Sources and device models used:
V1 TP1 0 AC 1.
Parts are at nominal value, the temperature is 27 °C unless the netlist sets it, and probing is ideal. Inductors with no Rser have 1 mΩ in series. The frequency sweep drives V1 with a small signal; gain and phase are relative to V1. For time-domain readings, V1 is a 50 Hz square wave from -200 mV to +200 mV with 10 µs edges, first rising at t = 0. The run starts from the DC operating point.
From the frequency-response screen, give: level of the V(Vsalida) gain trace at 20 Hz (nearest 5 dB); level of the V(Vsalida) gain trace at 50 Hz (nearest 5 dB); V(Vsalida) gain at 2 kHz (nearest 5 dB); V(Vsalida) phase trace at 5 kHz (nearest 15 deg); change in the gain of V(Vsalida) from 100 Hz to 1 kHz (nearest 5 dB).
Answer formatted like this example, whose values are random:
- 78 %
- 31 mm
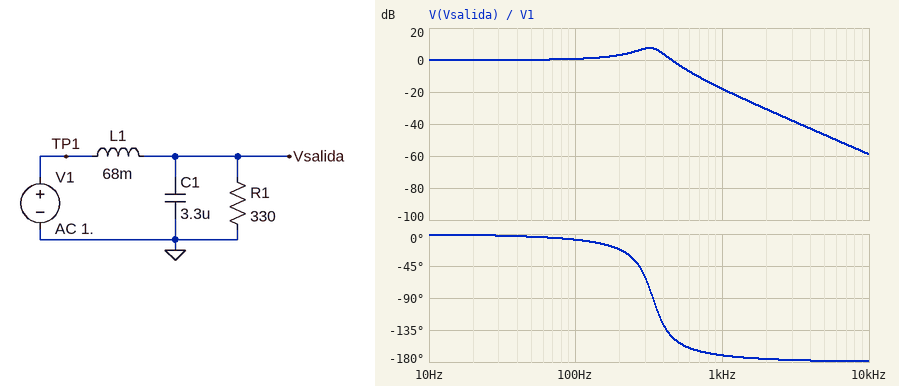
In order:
- 0 dB
- 0 dB
- -30 dB
- -180 deg
- -20 dB
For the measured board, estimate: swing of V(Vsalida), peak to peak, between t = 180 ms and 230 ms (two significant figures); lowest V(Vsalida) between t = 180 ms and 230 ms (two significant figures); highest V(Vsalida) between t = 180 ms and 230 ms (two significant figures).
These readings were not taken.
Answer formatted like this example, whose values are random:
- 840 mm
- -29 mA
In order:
- 800 mV
- -400 mV
- 400 mV
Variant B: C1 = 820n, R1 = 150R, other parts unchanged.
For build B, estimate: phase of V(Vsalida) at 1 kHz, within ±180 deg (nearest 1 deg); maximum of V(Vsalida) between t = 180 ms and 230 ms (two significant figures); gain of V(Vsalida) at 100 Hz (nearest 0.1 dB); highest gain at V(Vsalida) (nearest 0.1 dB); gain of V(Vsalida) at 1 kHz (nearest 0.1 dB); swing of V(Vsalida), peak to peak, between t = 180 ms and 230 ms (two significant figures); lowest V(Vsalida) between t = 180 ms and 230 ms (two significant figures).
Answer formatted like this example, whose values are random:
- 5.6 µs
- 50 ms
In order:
- -113 deg
- 200 mV
- -0.2 dB
- 0 dB
- -9.8 dB
- 400 mV
- -200 mV
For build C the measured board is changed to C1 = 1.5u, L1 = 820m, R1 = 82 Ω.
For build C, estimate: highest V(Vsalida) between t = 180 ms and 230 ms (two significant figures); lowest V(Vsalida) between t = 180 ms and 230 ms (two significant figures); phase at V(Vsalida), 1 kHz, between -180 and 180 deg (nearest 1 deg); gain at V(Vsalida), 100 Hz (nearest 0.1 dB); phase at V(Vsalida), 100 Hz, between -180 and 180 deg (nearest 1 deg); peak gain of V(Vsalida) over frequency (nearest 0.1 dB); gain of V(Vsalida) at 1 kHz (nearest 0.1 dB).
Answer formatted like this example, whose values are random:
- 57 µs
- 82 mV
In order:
- 92 mV
- -92 mV
- -127 deg
- -16.0 dB
- -85 deg
- 0 dB
- -37.9 dB
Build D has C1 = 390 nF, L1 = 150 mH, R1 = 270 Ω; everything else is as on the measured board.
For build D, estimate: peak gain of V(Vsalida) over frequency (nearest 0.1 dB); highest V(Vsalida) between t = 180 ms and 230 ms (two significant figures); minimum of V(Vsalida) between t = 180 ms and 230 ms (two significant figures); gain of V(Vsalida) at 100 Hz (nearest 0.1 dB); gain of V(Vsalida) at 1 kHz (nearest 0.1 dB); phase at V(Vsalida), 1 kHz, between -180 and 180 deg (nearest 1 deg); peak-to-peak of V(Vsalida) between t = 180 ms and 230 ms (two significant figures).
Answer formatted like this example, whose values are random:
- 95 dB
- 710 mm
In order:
- 0 dB
- 200 mV
- -200 mV
- -0.3 dB
- -11.4 dB
- -111 deg
- 400 mV
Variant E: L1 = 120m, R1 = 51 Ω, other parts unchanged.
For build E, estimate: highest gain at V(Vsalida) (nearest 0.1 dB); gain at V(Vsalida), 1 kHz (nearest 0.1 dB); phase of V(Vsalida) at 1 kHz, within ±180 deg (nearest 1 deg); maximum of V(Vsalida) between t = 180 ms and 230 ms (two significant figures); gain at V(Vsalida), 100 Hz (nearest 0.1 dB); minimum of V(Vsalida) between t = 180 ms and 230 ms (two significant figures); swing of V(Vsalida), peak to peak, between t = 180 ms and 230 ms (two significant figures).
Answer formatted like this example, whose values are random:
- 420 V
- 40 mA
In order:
- 0 dB
- -26.4 dB
- -135 deg
- 200 mV
- -4.6 dB
- -200 mV
- 390 mV
